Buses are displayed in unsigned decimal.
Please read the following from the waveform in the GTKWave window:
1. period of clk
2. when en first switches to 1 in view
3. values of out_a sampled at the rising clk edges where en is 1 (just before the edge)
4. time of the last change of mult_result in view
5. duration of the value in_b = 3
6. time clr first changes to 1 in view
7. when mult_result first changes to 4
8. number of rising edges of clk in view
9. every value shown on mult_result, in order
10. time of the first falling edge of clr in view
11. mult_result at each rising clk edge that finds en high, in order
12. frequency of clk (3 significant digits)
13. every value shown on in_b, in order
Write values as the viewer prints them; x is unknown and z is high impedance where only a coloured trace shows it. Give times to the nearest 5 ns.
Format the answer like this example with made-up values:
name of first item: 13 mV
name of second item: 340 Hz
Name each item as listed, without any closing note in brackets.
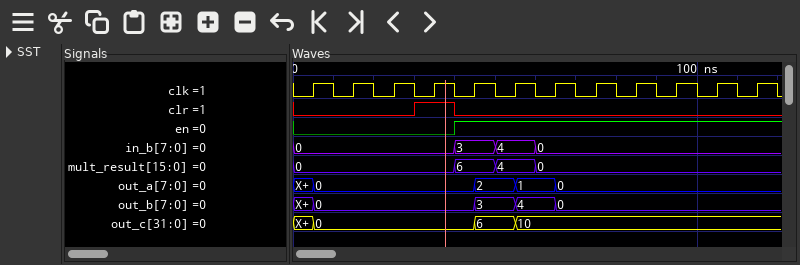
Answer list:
period of clk: 10 ns
when en first switches to 1 in view: 40 ns
values of out_a sampled at the rising clk edges where en is 1: 0, 2, 1, 0, 0, 0, 0, 0
time of the last change of mult_result in view: 60 ns
duration of the value in_b = 3: 10 ns
time clr first changes to 1 in view: 30 ns
when mult_result first changes to 4: 50 ns
number of rising edges of clk in view: 12
every value shown on mult_result, in order: 0, 6, 4, 0
time of the first falling edge of clr in view: 40 ns
mult_result at each rising clk edge that finds en high, in order: 6, 4, 0, 0, 0, 0, 0, 0
frequency of clk: 100 MHz
every value shown on in_b, in order: 0, 3, 4, 0
